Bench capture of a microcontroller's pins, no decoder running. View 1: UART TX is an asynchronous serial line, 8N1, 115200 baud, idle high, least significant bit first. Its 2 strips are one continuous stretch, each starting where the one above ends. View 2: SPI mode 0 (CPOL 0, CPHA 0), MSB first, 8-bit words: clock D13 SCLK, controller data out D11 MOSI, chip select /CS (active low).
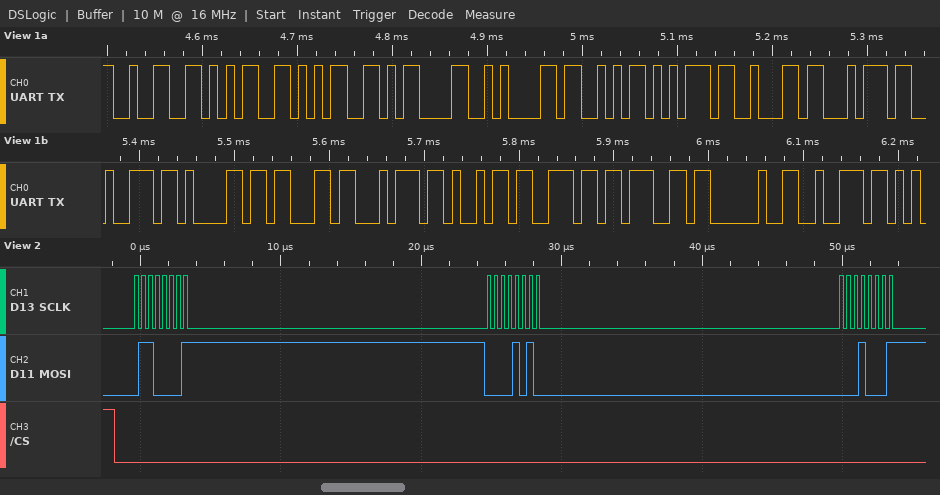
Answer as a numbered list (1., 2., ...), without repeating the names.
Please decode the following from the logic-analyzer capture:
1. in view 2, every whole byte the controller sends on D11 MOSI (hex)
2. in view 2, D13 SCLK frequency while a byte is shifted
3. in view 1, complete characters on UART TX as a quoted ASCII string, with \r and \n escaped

1. 61 0A 11
2. 2 MHz
3. "255\r\nSubtracting r"
